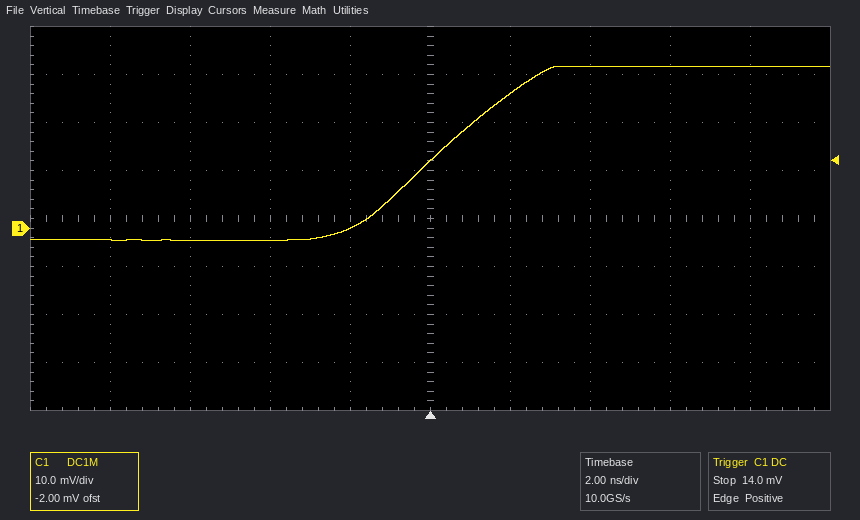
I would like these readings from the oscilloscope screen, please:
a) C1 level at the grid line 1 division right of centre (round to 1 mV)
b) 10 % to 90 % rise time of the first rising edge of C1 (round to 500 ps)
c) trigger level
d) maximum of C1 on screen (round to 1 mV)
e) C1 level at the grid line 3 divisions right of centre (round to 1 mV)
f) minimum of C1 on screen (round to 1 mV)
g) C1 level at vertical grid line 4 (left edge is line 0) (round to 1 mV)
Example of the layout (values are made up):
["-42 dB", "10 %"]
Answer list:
["28 mV", "4.0 ns", "14.0 mV", "34 mV", "34 mV", "-3 mV", "0 mV"]
